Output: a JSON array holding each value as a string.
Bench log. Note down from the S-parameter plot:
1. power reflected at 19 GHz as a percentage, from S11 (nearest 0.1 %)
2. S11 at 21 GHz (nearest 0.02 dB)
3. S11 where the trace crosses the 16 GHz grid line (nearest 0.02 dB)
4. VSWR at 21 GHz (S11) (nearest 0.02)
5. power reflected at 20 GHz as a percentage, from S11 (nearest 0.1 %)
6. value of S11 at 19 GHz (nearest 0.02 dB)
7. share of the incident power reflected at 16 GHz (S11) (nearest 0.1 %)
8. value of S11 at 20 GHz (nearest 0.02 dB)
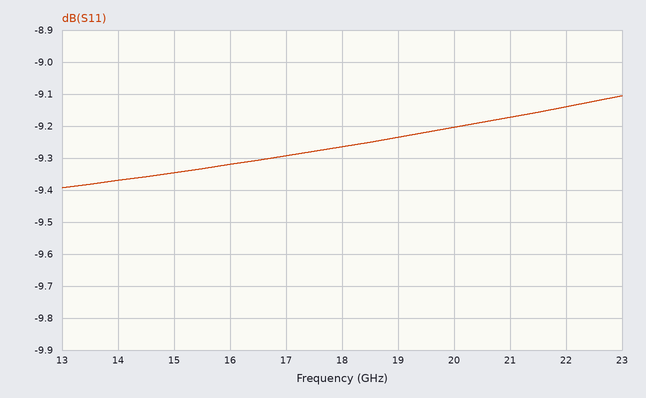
["11.9 %", "-9.18 dB", "-9.32 dB", "2.06", "12.0 %", "-9.24 dB", "11.7 %", "-9.20 dB"]
